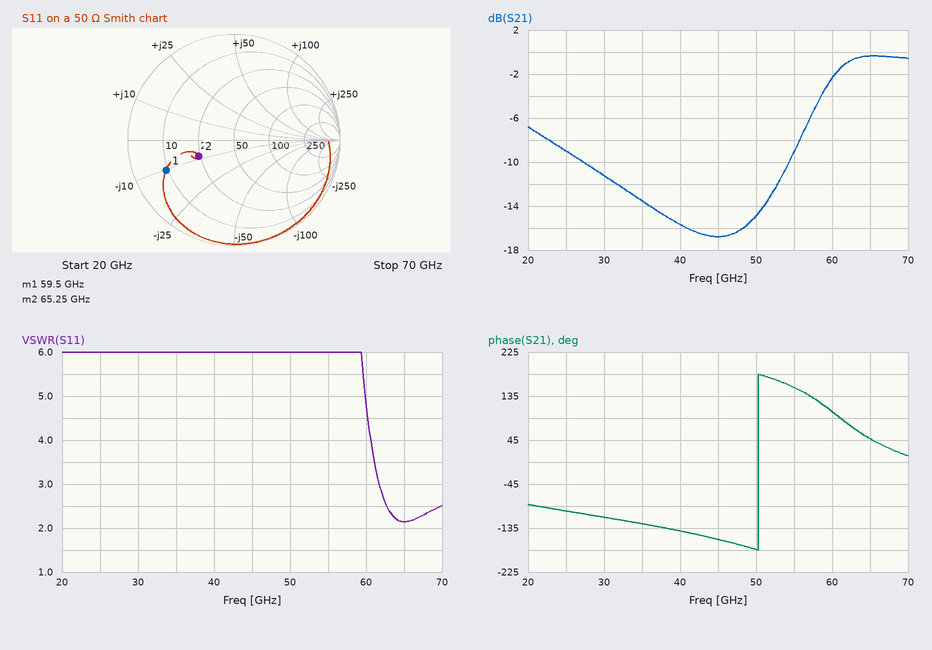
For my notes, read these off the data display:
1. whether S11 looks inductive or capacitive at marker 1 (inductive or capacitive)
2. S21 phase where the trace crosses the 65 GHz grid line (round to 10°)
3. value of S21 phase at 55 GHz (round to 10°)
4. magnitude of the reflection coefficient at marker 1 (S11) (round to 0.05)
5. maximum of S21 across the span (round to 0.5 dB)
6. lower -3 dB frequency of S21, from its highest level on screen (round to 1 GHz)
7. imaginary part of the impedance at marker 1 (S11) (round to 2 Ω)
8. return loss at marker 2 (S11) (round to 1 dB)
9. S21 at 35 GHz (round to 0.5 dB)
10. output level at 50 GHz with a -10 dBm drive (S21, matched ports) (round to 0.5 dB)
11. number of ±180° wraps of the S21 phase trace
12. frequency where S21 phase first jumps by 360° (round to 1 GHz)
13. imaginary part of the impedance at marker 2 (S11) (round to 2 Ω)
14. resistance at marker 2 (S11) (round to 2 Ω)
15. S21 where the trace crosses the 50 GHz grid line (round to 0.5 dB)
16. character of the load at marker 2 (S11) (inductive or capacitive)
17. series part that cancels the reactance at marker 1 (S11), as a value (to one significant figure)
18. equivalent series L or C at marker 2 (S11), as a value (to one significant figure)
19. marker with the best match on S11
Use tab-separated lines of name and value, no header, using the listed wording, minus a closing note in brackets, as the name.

whether S11 looks inductive or capacitive at marker 1	capacitive
S21 phase where the trace crosses the 65 GHz grid line	50°
value of S21 phase at 55 GHz	150°
magnitude of the reflection coefficient at marker 1 (S11)	0.70
maximum of S21 across the span	-0.5 dB
lower -3 dB frequency of S21, from its highest level on screen	59 GHz
imaginary part of the impedance at marker 1 (S11)	-10 Ω
return loss at marker 2 (S11)	9 dB
S21 at 35 GHz	-13.5 dB
output level at 50 GHz with a -10 dBm drive (S21, matched ports)	-25.0 dBm
number of ±180° wraps of the S21 phase trace	1
frequency where S21 phase first jumps by 360°	50 GHz
imaginary part of the impedance at marker 2 (S11)	-8 Ω
resistance at marker 2 (S11)	24 Ω
S21 where the trace crosses the 50 GHz grid line	-15.0 dB
character of the load at marker 2 (S11)	capacitive
series part that cancels the reactance at marker 1 (S11), as a value	30 pH
equivalent series L or C at marker 2 (S11), as a value	300 fF
marker with the best match on S11	marker 2
